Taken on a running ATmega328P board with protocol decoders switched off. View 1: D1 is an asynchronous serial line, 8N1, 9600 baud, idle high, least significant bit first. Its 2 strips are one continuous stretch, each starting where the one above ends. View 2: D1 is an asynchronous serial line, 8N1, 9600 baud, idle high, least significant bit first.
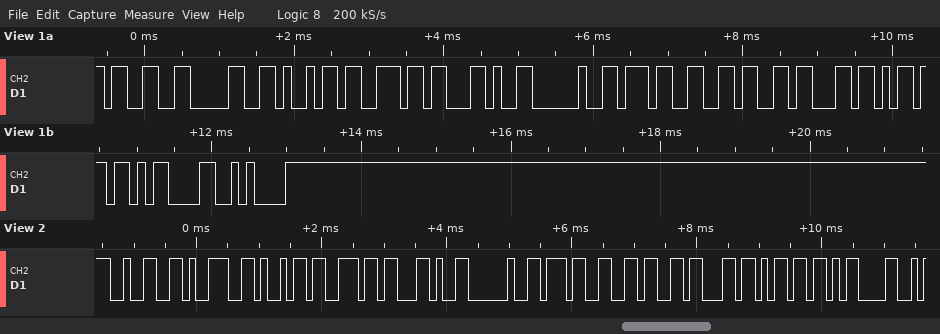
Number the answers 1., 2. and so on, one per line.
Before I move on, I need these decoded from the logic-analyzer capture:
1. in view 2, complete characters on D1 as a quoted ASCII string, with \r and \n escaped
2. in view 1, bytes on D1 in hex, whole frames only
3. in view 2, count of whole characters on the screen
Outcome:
1. "29in, 76cm\r"
2. 33 30 69 6E 2C 20 37 36 63 6D 0D 0A
3. 11
